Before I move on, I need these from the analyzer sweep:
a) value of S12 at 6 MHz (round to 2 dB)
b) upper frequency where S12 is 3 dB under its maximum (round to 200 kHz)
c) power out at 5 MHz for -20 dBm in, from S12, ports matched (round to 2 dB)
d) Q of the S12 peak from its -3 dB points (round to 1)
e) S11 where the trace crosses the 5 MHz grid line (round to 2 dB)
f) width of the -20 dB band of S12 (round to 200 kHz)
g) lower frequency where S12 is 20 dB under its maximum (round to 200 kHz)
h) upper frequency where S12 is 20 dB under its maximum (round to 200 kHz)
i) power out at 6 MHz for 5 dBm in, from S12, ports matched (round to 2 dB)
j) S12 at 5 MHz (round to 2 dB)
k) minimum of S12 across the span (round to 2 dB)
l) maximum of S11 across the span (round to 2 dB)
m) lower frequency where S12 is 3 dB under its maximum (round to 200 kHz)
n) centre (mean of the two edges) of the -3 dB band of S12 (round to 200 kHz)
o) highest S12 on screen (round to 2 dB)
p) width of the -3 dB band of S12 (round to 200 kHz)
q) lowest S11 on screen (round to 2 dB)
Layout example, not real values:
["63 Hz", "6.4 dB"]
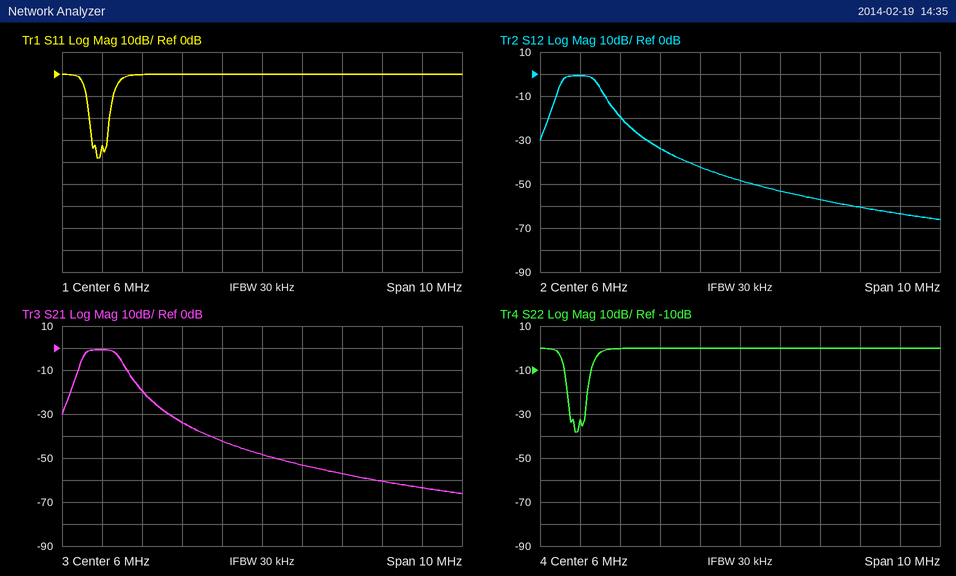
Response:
["-48 dB", "2.4 MHz", "-62 dBm", "2", "0 dB", "1.8 MHz", "1.2 MHz", "3.0 MHz", "-44 dBm", "-42 dB", "-66 dB", "0 dB", "1.6 MHz", "2.0 MHz", "0 dB", "800 kHz", "-38 dB"]
